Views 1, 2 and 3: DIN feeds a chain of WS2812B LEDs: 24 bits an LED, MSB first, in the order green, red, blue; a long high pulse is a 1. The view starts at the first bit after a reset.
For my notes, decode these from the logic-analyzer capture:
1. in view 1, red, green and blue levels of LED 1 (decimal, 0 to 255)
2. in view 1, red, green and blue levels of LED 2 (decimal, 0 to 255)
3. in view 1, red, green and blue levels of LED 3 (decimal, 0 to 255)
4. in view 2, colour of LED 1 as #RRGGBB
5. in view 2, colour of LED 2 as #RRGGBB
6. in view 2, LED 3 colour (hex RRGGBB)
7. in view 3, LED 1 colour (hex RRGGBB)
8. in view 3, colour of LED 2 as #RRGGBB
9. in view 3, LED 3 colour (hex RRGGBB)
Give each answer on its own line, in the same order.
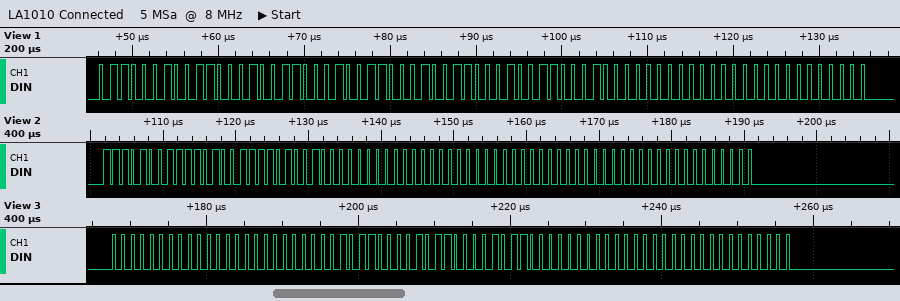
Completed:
98, 98, 98
98, 98, 98
0, 0, 0
#E9E9E9
#000000
#000000
#000000
#B0B0B0
#000000
